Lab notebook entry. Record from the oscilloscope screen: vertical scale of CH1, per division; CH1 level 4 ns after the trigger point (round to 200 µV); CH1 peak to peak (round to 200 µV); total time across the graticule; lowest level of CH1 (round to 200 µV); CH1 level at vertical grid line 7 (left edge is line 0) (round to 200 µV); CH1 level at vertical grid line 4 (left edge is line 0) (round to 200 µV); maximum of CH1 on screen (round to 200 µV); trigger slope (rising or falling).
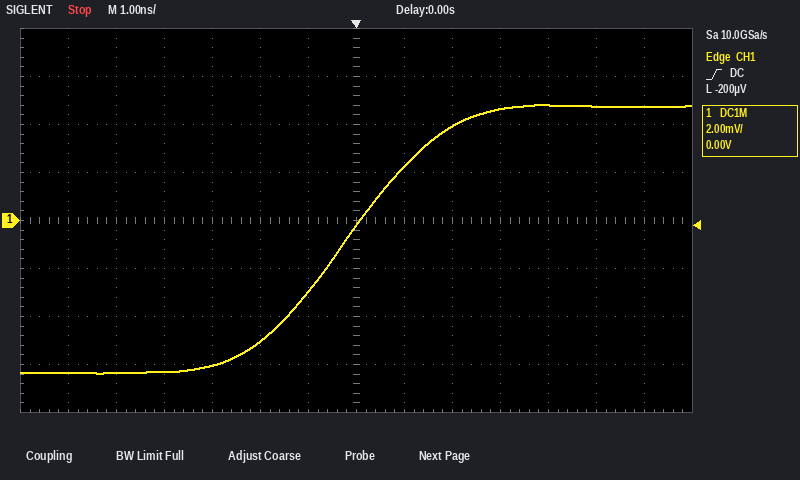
2 mV
4.8 mV
11.2 mV
14 ns
-6.4 mV
-200 µV
-6.0 mV
4.8 mV
rising
